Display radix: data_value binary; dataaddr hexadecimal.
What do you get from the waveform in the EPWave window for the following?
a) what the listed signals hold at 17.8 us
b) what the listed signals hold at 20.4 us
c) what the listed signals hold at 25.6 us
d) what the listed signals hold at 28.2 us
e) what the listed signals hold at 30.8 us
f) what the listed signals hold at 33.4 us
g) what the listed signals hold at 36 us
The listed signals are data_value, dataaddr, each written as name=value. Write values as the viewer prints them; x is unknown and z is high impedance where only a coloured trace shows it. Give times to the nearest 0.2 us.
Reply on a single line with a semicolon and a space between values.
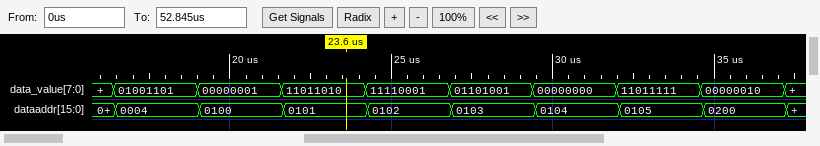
data_value=01001101, dataaddr=0004; data_value=00000001, dataaddr=0100; data_value=11110001, dataaddr=0102; data_value=01101001, dataaddr=0103; data_value=00000000, dataaddr=0104; data_value=11011111, dataaddr=0105; data_value=00000010, dataaddr=0200
